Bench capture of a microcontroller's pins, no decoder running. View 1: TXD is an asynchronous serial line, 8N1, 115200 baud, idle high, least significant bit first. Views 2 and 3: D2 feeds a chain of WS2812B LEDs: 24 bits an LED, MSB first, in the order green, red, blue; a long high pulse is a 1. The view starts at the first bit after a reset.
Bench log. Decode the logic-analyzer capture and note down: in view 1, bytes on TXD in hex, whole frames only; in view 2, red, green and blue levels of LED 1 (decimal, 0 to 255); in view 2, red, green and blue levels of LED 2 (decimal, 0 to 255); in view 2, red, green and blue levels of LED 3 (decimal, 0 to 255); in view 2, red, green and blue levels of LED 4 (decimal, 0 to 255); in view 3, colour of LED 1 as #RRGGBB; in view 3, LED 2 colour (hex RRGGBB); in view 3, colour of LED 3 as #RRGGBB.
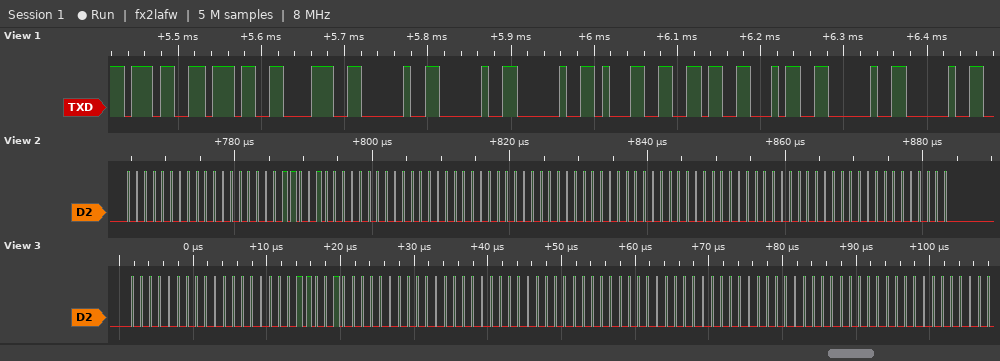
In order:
37 37 38 20 20 20 31 36 34 20 20
0, 0, 50
0, 0, 0
0, 0, 0
0, 0, 0
#000032
#000000
#000000
